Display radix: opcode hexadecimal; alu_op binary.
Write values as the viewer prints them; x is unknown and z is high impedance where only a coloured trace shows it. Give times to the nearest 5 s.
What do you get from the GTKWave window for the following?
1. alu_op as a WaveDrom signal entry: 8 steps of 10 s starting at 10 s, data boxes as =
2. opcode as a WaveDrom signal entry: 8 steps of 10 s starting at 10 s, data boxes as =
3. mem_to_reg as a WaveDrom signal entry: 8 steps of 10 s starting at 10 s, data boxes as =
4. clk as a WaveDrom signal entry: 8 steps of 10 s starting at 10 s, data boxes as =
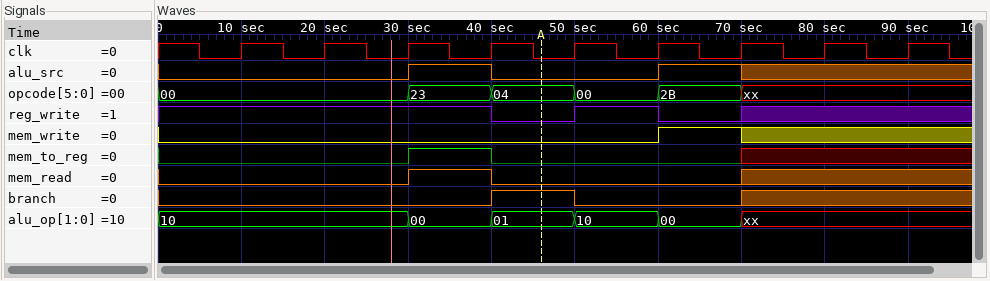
{name: 'alu_op', wave: '=.====x.', data: '10 00 01 10 00'}
{name: 'opcode', wave: '=.====x.', data: '00 23 04 00 2B'}
{name: 'mem_to_reg', wave: '0.10..x.'}
{name: 'clk', wave: 'p.......'}
